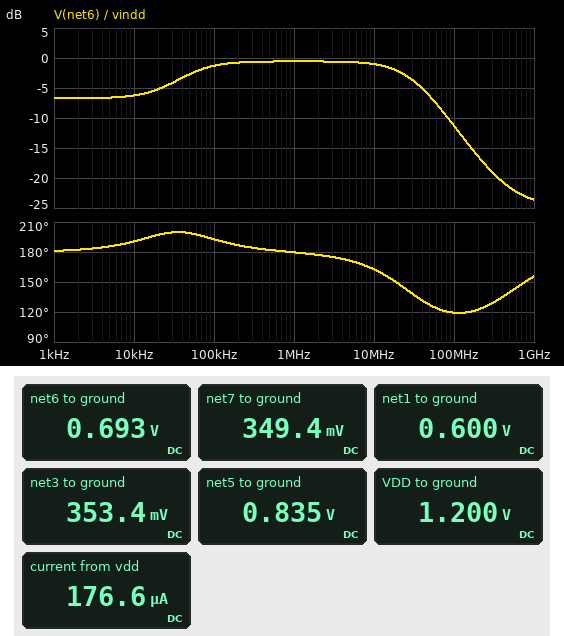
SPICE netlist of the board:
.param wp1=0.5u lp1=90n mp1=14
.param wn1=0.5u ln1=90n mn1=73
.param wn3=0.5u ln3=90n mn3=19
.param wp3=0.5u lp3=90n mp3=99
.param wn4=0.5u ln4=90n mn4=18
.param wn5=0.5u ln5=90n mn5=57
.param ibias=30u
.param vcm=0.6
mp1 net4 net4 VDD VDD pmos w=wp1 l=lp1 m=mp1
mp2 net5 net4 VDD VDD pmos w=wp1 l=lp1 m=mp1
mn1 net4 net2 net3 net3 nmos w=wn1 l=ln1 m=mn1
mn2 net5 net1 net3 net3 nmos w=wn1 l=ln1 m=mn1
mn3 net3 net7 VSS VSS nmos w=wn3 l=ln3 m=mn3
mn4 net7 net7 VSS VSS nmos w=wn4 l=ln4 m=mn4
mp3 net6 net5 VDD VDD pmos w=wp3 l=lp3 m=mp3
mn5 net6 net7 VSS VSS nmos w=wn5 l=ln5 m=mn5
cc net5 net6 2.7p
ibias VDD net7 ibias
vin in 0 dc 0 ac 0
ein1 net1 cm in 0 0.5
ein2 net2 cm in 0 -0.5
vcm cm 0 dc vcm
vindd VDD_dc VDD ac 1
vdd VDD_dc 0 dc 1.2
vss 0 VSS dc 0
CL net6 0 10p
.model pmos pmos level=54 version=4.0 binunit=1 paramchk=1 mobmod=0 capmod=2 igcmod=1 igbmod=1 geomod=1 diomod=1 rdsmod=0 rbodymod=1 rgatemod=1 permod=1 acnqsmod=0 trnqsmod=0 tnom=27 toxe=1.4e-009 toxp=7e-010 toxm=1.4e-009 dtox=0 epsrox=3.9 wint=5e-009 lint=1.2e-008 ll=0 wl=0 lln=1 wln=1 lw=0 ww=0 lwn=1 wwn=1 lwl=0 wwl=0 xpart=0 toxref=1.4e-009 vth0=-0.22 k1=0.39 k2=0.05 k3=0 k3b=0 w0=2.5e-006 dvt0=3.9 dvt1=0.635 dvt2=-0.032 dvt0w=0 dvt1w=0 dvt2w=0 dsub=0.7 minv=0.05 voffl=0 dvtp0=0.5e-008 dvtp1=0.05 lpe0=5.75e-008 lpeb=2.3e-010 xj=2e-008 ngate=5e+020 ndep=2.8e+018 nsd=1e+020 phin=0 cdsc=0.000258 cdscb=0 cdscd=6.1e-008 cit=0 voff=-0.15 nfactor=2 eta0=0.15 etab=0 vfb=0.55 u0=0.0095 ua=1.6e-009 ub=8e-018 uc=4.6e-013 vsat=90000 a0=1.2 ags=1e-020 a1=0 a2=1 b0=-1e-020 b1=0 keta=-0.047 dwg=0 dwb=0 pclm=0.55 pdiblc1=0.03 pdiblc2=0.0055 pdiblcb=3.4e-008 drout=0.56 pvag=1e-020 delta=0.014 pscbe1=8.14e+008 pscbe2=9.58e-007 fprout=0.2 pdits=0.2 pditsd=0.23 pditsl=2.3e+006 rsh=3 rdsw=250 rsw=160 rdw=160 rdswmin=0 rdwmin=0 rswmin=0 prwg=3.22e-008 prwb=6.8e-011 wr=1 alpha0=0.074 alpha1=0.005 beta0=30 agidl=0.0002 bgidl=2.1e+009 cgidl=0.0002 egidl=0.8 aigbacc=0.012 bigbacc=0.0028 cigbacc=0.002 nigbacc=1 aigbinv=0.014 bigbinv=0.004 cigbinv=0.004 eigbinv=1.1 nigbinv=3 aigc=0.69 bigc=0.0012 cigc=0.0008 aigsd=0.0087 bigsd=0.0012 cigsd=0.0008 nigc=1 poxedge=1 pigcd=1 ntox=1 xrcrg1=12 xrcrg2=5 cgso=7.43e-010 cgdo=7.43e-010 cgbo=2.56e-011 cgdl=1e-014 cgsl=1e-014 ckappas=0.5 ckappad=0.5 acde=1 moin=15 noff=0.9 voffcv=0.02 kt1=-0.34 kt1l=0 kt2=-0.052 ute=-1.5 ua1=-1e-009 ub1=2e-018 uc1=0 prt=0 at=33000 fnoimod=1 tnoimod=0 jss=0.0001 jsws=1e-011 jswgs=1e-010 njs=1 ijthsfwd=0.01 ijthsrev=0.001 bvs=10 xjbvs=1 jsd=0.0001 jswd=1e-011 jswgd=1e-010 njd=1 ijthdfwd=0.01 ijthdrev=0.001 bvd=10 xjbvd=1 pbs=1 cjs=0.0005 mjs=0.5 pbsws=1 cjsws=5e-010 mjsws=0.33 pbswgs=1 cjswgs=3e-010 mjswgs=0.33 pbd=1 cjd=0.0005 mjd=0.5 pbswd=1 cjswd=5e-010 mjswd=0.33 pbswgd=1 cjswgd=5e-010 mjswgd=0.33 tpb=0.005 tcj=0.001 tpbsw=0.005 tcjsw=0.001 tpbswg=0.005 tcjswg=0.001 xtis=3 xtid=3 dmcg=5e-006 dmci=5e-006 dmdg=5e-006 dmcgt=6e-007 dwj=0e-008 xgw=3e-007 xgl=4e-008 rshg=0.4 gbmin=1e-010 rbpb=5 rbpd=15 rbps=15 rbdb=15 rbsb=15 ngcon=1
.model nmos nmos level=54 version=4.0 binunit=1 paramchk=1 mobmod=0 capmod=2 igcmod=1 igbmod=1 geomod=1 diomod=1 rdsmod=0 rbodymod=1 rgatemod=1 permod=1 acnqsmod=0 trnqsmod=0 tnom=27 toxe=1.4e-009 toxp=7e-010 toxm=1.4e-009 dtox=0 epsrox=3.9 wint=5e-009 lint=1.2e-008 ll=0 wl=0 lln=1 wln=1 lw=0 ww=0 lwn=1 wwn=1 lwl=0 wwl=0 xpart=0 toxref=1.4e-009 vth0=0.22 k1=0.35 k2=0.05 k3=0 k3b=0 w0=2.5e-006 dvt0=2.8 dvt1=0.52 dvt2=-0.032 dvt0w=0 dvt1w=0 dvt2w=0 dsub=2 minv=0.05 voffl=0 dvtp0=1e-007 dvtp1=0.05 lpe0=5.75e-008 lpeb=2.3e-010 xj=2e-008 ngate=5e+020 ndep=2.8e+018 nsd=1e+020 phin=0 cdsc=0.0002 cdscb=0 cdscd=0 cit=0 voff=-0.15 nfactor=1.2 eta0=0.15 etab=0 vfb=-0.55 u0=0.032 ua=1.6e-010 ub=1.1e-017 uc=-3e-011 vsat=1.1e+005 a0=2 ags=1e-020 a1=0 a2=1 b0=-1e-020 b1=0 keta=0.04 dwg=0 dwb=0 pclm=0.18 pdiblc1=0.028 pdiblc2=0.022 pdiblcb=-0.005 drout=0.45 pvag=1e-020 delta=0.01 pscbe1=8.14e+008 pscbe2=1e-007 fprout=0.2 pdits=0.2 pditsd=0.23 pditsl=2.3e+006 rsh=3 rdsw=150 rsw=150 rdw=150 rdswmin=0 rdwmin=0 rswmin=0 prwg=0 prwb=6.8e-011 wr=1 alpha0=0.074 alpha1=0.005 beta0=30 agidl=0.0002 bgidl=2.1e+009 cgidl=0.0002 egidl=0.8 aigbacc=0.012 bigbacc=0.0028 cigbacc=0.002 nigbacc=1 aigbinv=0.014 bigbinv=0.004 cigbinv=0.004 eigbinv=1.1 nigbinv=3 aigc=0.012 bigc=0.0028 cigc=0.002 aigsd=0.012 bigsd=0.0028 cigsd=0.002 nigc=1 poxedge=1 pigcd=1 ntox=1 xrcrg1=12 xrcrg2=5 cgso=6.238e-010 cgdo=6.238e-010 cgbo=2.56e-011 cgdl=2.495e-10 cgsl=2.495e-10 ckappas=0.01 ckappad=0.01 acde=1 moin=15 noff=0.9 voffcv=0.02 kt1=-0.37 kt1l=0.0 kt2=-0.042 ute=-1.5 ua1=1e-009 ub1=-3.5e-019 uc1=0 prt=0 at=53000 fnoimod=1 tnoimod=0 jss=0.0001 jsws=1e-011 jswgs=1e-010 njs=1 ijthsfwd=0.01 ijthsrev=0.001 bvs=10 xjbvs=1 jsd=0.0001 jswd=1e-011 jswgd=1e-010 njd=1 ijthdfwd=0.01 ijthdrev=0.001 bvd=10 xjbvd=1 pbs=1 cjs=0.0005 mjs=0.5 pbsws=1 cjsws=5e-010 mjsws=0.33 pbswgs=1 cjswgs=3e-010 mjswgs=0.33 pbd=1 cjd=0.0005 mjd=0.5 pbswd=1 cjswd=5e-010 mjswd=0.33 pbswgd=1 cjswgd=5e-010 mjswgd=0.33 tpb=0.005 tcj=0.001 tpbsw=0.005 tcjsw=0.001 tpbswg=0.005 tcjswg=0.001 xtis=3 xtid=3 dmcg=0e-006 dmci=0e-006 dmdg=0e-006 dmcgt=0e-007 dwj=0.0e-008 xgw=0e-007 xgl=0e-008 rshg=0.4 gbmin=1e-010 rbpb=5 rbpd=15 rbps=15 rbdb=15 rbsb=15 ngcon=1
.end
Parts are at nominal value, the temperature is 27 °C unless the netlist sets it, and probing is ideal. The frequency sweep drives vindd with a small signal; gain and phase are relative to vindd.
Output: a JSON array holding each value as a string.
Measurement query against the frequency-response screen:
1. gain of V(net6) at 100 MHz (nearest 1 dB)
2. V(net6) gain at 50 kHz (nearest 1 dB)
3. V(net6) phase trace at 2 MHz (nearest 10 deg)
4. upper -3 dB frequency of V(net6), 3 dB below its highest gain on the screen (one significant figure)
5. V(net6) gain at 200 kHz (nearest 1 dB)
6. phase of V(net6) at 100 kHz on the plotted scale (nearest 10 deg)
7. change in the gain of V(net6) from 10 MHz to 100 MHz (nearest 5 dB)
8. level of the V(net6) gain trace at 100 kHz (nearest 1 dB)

["-11 dB", "-3 dB", "180 deg", "30 MHz", "-1 dB", "190 deg", "-10 dB", "-1 dB"]
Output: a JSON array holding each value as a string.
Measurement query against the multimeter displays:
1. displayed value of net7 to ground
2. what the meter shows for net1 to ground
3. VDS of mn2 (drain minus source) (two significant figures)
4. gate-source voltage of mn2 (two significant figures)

["349.4 mV", "0.600 V", "480 mV", "250 mV"]
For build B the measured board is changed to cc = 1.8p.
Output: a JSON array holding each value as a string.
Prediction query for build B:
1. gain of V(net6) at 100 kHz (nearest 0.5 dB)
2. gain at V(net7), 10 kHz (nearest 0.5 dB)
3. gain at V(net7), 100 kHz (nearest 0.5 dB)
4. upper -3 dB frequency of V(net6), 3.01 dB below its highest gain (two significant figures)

["-2.0 dB", "-61.5 dB", "-57.0 dB", "29 MHz"]
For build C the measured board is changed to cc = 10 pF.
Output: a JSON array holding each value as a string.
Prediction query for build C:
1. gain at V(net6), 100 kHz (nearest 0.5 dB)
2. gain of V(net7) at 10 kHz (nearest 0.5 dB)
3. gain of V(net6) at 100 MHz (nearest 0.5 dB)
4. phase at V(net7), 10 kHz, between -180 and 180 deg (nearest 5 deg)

["-0.5 dB", "-58.5 dB", "-11.0 dB", "-160 deg"]
